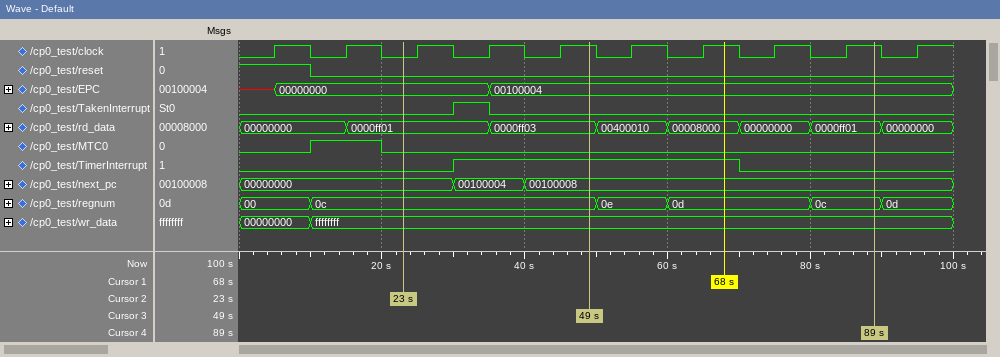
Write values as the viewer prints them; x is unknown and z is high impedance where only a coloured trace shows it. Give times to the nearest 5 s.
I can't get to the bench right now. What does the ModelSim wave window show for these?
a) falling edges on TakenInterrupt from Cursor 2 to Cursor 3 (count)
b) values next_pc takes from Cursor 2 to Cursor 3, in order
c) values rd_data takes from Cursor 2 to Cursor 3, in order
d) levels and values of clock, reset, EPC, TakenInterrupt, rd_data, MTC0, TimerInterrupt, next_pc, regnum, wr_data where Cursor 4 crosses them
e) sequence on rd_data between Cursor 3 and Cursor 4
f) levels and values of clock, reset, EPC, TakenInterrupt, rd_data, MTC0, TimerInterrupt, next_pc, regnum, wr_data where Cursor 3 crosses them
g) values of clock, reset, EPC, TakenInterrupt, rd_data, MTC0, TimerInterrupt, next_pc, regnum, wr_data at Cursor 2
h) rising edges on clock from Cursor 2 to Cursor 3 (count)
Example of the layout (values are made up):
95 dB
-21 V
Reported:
1
00000000, 00100004, 00100008
0000ff01, 0000ff03
clock=1, reset=0, EPC=00100004, TakenInterrupt=0, rd_data=0000ff01, MTC0=0, TimerInterrupt=0, next_pc=00100008, regnum=0c, wr_data=ffffffff
0000ff03, 00400010, 00008000, 00000000, 0000ff01
clock=1, reset=0, EPC=00100004, TakenInterrupt=0, rd_data=0000ff03, MTC0=0, TimerInterrupt=1, next_pc=00100008, regnum=0c, wr_data=ffffffff
clock=0, reset=0, EPC=00000000, TakenInterrupt=0, rd_data=0000ff01, MTC0=0, TimerInterrupt=0, next_pc=00000000, regnum=0c, wr_data=ffffffff
3
